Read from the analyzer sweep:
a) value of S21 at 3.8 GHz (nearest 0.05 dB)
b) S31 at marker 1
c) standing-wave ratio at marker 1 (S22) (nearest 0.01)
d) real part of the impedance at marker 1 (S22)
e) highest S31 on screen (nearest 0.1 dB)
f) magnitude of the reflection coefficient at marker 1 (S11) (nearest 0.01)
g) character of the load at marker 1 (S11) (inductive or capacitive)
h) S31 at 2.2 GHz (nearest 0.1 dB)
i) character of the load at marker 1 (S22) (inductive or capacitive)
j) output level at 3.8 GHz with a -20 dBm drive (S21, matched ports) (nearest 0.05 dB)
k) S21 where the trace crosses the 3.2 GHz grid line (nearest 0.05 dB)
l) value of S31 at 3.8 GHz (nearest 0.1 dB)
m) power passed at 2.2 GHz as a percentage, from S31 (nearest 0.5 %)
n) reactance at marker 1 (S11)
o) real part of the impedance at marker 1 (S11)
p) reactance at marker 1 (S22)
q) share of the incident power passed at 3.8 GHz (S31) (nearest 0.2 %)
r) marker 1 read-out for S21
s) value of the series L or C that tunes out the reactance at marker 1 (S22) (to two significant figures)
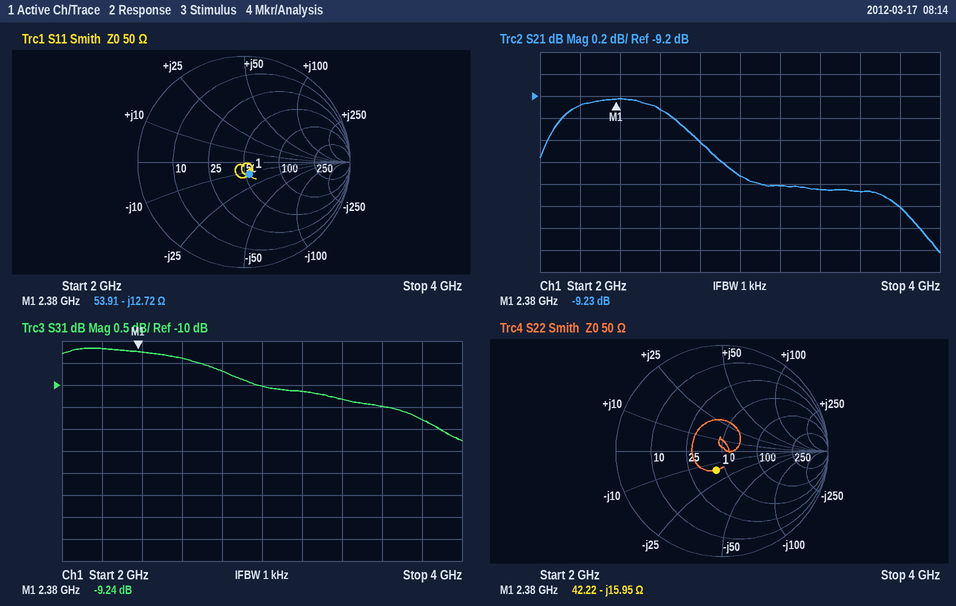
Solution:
-10.20 dB
-9.24 dB
1.47
42.22 Ω
-9.2 dB
0.13
capacitive
-9.2 dB
capacitive
-30.20 dBm
-10.00 dB
-10.8 dB
12.0 %
-12.72 Ω
53.91 Ω
-15.95 Ω
8.4 %
-9.23 dB
1.1 nH
